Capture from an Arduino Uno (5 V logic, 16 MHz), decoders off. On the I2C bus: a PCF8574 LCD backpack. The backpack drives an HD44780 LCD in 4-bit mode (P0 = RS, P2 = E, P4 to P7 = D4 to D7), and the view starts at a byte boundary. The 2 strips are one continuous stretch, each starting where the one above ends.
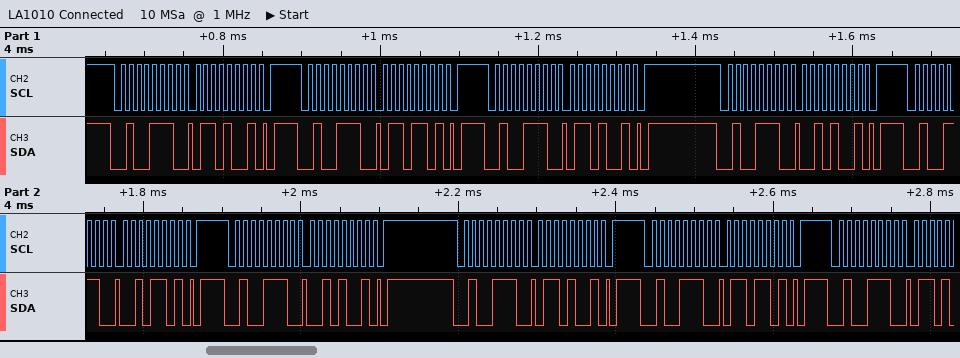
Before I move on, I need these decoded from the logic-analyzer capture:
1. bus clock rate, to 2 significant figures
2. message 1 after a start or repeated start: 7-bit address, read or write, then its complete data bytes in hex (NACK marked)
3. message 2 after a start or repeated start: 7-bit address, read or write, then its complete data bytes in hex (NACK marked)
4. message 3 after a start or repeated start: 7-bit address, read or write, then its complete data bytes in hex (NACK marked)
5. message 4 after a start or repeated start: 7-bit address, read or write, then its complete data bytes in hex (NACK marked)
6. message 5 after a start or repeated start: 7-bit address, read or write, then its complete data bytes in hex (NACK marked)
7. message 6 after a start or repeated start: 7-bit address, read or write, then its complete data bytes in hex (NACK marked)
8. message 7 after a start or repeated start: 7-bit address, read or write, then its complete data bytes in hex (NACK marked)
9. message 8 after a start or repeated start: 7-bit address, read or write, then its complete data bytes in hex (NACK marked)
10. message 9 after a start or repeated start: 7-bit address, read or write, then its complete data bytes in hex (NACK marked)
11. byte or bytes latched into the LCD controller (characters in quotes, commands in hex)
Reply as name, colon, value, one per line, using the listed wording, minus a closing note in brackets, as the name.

bus clock rate, to 2 significant figures: 100 kHz
message 1 after a start or repeated start: 7-bit address, read or write, then its complete data bytes in hex: 0x27 write: 69
message 2 after a start or repeated start: 7-bit address, read or write, then its complete data bytes in hex: 0x27 write: 6D
message 3 after a start or repeated start: 7-bit address, read or write, then its complete data bytes in hex: 0x27 write: 69
message 4 after a start or repeated start: 7-bit address, read or write, then its complete data bytes in hex: 0x27 write: 29
message 5 after a start or repeated start: 7-bit address, read or write, then its complete data bytes in hex: 0x27 write: 2D
message 6 after a start or repeated start: 7-bit address, read or write, then its complete data bytes in hex: 0x27 write: 29
message 7 after a start or repeated start: 7-bit address, read or write, then its complete data bytes in hex: 0x27 write: 69
message 8 after a start or repeated start: 7-bit address, read or write, then its complete data bytes in hex: 0x27 write: 6D
message 9 after a start or repeated start: 7-bit address, read or write, then its complete data bytes in hex: 0x27 write
byte or bytes latched into the LCD controller: 'b'
